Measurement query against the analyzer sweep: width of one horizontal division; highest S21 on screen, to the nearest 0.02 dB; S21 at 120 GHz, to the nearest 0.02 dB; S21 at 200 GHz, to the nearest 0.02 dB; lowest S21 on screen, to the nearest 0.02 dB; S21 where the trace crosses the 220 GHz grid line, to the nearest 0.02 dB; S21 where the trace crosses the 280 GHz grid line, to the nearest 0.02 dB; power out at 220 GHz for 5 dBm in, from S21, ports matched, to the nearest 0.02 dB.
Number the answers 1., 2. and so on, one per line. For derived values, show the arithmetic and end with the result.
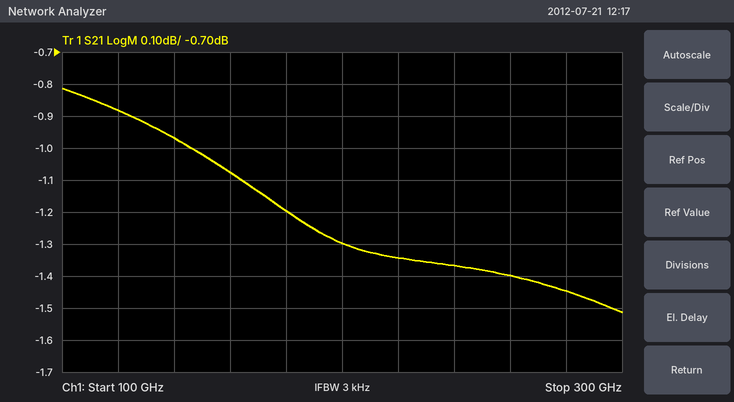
1. 20 GHz
2. -0.82 dB
3. -0.88 dB
4. -1.30 dB
5. -1.52 dB
6. -1.34 dB
7. -1.44 dB
8. 5 dBm + (-1.34 dB) = 3.66 dBm
